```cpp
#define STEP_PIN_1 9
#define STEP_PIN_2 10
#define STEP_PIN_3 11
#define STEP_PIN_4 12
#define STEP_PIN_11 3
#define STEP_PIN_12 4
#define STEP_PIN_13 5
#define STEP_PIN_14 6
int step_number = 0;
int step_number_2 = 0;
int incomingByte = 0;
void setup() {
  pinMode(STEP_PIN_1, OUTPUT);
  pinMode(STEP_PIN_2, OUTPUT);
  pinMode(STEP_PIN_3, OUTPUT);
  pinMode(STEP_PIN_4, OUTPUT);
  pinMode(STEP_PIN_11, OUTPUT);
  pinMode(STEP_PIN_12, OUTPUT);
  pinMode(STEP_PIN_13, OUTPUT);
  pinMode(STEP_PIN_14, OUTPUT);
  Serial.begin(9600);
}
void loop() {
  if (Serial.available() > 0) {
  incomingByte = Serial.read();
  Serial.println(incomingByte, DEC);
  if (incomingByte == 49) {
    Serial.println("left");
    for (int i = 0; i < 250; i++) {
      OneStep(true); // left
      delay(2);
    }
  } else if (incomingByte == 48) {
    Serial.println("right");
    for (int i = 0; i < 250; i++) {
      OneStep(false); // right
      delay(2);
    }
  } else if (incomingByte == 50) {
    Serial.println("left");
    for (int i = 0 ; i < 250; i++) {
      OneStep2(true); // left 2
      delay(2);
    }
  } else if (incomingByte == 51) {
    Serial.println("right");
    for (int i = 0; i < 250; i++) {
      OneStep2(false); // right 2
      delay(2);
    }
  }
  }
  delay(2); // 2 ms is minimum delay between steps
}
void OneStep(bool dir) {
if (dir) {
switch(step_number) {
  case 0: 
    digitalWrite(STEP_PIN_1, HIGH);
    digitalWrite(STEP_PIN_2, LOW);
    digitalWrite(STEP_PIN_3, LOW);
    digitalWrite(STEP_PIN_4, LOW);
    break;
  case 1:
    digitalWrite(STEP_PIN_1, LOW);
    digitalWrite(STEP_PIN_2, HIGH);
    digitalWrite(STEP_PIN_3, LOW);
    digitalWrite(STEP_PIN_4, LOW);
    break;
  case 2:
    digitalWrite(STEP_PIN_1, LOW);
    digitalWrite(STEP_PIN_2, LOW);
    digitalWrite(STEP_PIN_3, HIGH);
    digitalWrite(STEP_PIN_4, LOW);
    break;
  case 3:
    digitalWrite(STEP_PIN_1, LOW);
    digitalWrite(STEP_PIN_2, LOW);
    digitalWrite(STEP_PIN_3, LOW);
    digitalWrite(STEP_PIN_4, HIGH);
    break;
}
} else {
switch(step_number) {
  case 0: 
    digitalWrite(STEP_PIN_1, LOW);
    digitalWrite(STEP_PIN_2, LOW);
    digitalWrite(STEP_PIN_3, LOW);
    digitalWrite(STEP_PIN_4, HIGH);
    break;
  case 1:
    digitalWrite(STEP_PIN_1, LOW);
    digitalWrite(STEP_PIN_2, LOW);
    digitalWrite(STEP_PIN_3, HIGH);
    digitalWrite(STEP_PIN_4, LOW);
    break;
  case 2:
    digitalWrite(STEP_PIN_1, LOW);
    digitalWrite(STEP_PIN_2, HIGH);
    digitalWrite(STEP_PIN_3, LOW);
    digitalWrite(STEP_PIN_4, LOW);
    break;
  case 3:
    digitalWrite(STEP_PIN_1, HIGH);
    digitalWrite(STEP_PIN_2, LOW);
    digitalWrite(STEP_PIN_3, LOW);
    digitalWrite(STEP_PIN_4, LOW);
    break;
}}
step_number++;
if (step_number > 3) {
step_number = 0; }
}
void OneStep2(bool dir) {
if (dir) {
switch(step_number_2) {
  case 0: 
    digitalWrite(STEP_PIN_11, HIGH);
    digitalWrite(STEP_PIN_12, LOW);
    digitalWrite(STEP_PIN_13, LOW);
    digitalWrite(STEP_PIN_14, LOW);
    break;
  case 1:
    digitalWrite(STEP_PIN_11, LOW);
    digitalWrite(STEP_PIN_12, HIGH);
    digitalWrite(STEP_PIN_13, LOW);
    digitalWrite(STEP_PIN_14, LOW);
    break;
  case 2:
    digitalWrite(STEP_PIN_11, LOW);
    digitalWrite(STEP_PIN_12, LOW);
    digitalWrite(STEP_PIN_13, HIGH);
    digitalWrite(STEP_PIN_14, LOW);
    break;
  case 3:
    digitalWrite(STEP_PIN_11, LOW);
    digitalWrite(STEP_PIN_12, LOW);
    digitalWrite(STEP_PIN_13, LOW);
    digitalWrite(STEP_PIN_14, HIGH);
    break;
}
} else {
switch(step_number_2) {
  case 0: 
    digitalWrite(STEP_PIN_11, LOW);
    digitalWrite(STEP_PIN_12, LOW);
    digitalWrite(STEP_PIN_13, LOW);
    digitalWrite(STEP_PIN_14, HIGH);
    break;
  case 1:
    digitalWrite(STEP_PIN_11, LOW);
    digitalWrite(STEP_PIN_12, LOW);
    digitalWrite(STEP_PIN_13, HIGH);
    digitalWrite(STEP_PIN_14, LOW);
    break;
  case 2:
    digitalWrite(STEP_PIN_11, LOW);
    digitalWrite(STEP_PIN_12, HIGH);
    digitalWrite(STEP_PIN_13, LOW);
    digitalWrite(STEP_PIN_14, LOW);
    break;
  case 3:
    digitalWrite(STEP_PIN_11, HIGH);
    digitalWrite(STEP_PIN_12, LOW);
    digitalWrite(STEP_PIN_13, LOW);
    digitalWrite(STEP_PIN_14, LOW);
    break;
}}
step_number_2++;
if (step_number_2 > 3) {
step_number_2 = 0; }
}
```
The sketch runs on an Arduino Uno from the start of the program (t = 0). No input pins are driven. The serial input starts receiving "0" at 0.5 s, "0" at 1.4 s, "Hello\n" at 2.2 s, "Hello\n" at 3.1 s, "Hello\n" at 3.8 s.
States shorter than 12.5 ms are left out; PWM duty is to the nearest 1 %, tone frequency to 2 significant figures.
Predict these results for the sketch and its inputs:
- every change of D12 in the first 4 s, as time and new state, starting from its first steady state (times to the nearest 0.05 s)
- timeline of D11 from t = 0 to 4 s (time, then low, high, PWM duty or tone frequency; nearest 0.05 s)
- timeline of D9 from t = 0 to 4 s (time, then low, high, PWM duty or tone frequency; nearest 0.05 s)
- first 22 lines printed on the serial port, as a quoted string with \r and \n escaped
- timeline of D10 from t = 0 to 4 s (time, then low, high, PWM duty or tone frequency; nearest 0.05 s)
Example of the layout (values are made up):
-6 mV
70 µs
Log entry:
0 s low; 0.5 s tone 120 Hz; 1 s low; 1.4 s tone 120 Hz; 1.9 s low
0 s low; 0.5 s tone 120 Hz; 1 s high; 1.4 s tone 120 Hz; 1.9 s low
0 s low; 0.5 s tone 120 Hz; 1 s low; 1.4 s tone 120 Hz; 1.9 s high
"48\r\nright\r\n48\r\nright\r\n72\r\n101\r\n108\r\n108\r\n111\r\n10\r\n72\r\n101\r\n108\r\n108\r\n111\r\n10\r\n72\r\n101\r\n108\r\n108\r\n111\r\n10\r\n"
0 s low; 0.5 s tone 120 Hz; 1 s low; 1.4 s tone 120 Hz; 1.9 s low
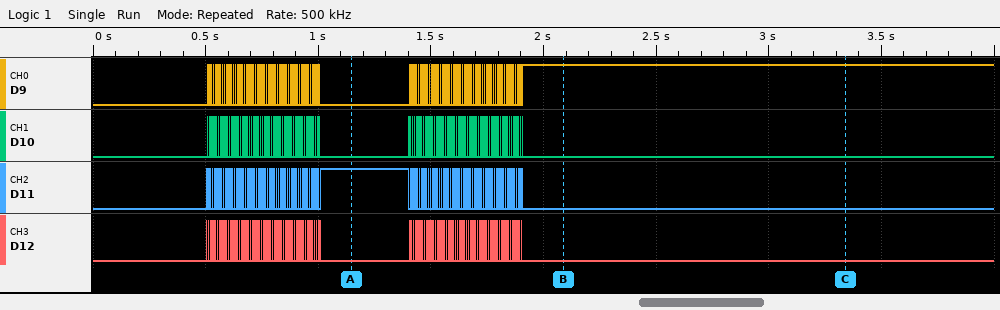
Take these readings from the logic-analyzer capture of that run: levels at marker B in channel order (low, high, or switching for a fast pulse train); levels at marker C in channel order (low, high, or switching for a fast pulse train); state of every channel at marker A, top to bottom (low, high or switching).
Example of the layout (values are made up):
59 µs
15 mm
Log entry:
D9 high, D10 low, D11 low, D12 low
D9 high, D10 low, D11 low, D12 low
D9 low, D10 low, D11 high, D12 low
